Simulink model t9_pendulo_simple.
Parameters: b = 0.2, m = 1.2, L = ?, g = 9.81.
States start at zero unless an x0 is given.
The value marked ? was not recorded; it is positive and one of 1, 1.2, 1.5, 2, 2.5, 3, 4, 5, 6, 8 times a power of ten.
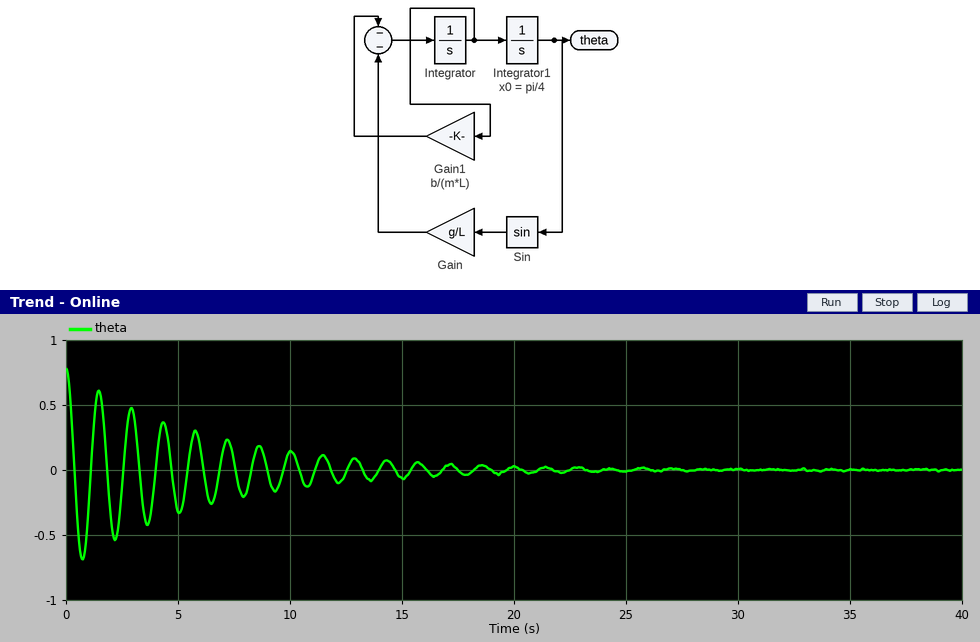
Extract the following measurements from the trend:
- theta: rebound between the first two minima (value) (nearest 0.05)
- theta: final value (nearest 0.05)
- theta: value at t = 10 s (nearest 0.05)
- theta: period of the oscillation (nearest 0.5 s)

0.60
0.00
0.15
1.5 s
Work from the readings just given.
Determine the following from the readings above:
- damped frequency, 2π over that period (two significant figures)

4.2 rad/s
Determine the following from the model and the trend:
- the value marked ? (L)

0.5
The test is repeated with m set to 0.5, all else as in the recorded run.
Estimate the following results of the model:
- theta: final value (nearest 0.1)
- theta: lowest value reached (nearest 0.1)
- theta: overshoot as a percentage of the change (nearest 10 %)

0.0
-0.6
70 %
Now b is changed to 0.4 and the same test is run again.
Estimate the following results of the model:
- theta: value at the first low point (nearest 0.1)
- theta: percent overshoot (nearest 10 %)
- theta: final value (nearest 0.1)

-0.6
80 %
0.0
